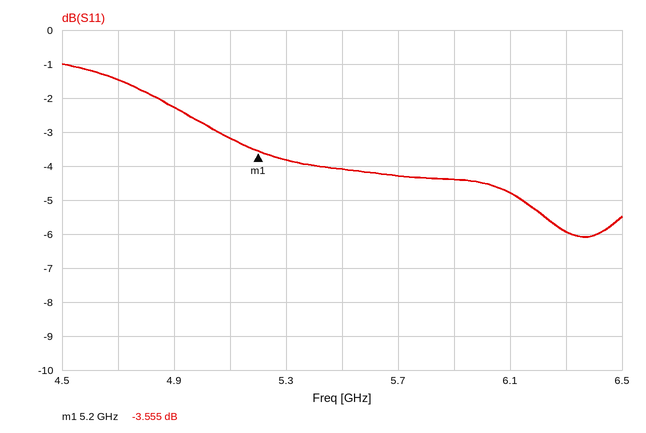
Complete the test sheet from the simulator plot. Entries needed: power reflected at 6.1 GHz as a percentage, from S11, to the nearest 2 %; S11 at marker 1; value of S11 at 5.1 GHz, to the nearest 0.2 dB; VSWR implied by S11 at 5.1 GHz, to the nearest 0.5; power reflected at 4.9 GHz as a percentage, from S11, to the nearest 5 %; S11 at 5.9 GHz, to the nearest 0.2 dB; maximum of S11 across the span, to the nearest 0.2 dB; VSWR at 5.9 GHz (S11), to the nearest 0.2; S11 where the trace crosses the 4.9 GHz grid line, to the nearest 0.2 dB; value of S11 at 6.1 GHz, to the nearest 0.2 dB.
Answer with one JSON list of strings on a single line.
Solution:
["34 %", "-3.555 dB", "-3.2 dB", "5.5", "60 %", "-4.4 dB", "-1.0 dB", "4.0", "-2.2 dB", "-4.8 dB"]
